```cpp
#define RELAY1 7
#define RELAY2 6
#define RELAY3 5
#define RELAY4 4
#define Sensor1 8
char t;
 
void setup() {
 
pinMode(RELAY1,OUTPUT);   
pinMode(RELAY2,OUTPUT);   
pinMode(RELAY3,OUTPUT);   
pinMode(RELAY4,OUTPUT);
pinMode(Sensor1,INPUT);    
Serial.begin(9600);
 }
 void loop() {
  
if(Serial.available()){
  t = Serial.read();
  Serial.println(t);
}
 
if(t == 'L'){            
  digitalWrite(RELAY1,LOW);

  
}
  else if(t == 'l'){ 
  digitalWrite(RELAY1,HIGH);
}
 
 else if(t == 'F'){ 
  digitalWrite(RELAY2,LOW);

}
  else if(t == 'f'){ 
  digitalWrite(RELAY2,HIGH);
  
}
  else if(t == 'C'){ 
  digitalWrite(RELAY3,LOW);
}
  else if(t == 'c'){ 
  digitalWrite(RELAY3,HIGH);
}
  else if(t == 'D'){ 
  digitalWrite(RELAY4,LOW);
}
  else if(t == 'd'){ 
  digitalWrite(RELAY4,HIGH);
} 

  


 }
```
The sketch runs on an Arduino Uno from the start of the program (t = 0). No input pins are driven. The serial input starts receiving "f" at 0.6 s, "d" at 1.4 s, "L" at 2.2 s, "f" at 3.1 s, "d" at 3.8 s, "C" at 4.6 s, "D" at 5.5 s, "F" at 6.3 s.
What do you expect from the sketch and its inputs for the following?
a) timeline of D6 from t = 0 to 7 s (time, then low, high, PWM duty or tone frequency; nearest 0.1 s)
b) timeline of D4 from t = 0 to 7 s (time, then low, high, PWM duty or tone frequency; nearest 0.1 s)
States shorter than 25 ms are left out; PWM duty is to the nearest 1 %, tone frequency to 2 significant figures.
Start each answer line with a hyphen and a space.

- 0 s low; 0.6 s high; 6.3 s low
- 0 s low; 1.4 s high; 5.5 s low
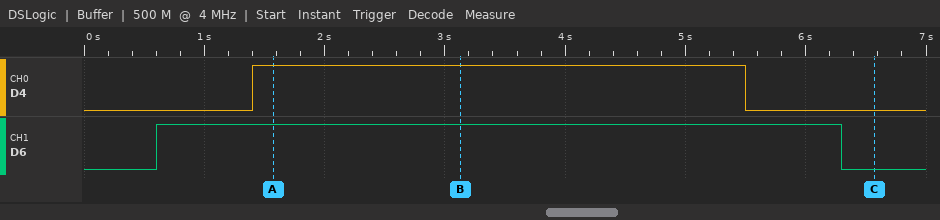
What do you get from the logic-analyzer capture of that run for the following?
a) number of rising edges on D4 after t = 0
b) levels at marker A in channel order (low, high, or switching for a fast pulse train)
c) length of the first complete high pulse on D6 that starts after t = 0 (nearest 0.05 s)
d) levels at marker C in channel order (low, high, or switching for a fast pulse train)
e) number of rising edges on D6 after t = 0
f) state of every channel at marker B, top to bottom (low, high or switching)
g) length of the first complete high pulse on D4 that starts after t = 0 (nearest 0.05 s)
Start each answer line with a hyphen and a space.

- 1
- D4 high, D6 high
- 5.70 s
- D4 low, D6 low
- 1
- D4 high, D6 high
- 4.10 s
